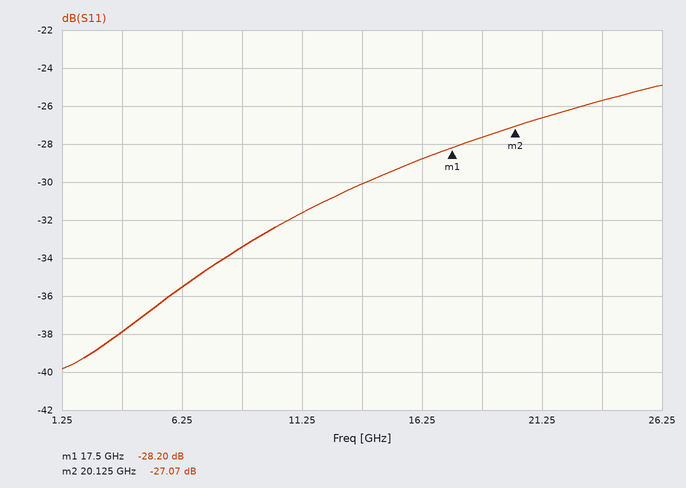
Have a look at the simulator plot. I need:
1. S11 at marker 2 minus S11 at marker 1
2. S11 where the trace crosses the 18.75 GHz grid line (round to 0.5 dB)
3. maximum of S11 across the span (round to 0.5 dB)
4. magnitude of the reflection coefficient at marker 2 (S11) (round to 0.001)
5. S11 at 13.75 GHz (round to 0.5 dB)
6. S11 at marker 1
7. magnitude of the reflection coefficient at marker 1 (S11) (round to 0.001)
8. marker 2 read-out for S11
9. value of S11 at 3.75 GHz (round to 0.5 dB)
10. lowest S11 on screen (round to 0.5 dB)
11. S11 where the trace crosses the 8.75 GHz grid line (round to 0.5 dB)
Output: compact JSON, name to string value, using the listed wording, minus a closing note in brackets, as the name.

{"S11 at marker 2 minus S11 at marker 1": "1.13 dB", "S11 where the trace crosses the 18.75 GHz grid line": "-27.5 dB", "maximum of S11 across the span": "-25.0 dB", "magnitude of the reflection coefficient at marker 2 (S11)": "0.044", "S11 at 13.75 GHz": "-30.0 dB", "S11 at marker 1": "-28.20 dB", "magnitude of the reflection coefficient at marker 1 (S11)": "0.039", "marker 2 read-out for S11": "-27.07 dB", "value of S11 at 3.75 GHz": "-38.0 dB", "lowest S11 on screen": "-40.0 dB", "S11 where the trace crosses the 8.75 GHz grid line": "-33.5 dB"}
